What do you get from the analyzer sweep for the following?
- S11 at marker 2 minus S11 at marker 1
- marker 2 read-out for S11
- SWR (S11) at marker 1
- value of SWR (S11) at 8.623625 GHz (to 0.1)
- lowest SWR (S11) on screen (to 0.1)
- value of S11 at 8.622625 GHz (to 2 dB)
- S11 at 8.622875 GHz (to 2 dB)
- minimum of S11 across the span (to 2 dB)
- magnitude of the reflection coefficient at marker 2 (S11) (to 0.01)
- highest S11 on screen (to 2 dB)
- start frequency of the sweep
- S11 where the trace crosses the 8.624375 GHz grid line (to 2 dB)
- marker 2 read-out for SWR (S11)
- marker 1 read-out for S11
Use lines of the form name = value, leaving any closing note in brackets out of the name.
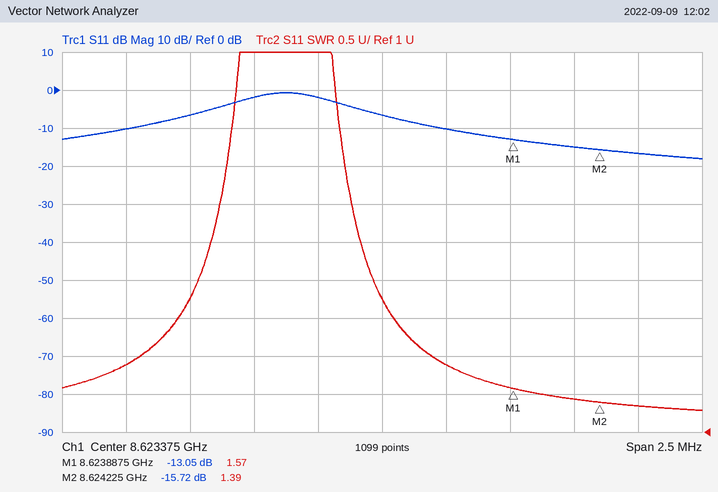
S11 at marker 2 minus S11 at marker 1 = -2.67 dB
marker 2 read-out for S11 = -15.72 dB
SWR (S11) at marker 1 = 1.57
value of SWR (S11) at 8.623625 GHz = 1.9
lowest SWR (S11) on screen = 1.3
value of S11 at 8.622625 GHz = -6 dB
S11 at 8.622875 GHz = -2 dB
minimum of S11 across the span = -18 dB
magnitude of the reflection coefficient at marker 2 (S11) = 0.16
highest S11 on screen = 0 dB
start frequency of the sweep = 8.622125 GHz
S11 where the trace crosses the 8.624375 GHz grid line = -16 dB
marker 2 read-out for SWR = 1.39
marker 1 read-out for S11 = -13.05 dB
